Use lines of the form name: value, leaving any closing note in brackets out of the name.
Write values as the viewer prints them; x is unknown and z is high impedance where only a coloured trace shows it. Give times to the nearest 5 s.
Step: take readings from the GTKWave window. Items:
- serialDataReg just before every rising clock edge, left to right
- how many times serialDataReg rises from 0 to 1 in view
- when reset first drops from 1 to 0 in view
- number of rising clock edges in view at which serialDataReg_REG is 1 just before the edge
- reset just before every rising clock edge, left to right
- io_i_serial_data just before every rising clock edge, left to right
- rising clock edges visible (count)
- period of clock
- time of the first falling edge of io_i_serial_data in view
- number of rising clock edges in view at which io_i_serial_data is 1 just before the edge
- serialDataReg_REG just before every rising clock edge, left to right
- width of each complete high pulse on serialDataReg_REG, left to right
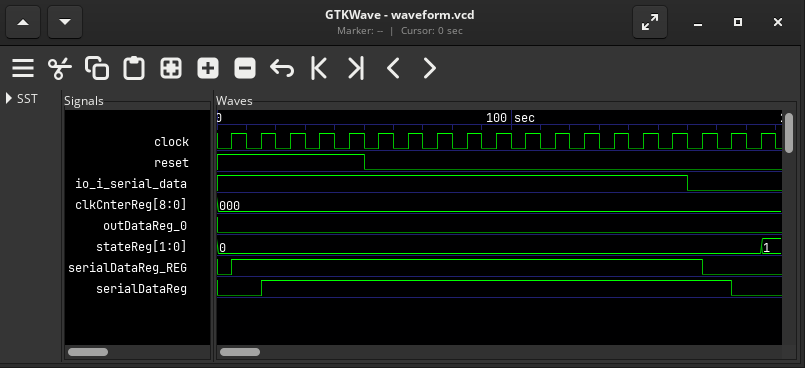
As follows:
serialDataReg just before every rising clock edge, left to right: 0 0 1 1 1 1 1 1 1 1 1 1 1 1 1 1 1 1 0
how many times serialDataReg rises from 0 to 1 in view: 1
when reset first drops from 1 to 0 in view: 50 s
number of rising clock edges in view at which serialDataReg_REG is 1 just before the edge: 16
reset just before every rising clock edge, left to right: 1 1 1 1 1 0 0 0 0 0 0 0 0 0 0 0 0 0 0
io_i_serial_data just before every rising clock edge, left to right: 1 1 1 1 1 1 1 1 1 1 1 1 1 1 1 1 0 0 0
rising clock edges visible: 19
period of clock: 10 s
time of the first falling edge of io_i_serial_data in view: 160 s
number of rising clock edges in view at which io_i_serial_data is 1 just before the edge: 16
serialDataReg_REG just before every rising clock edge, left to right: 0 1 1 1 1 1 1 1 1 1 1 1 1 1 1 1 1 0 0
width of each complete high pulse on serialDataReg_REG, left to right: 160 s
